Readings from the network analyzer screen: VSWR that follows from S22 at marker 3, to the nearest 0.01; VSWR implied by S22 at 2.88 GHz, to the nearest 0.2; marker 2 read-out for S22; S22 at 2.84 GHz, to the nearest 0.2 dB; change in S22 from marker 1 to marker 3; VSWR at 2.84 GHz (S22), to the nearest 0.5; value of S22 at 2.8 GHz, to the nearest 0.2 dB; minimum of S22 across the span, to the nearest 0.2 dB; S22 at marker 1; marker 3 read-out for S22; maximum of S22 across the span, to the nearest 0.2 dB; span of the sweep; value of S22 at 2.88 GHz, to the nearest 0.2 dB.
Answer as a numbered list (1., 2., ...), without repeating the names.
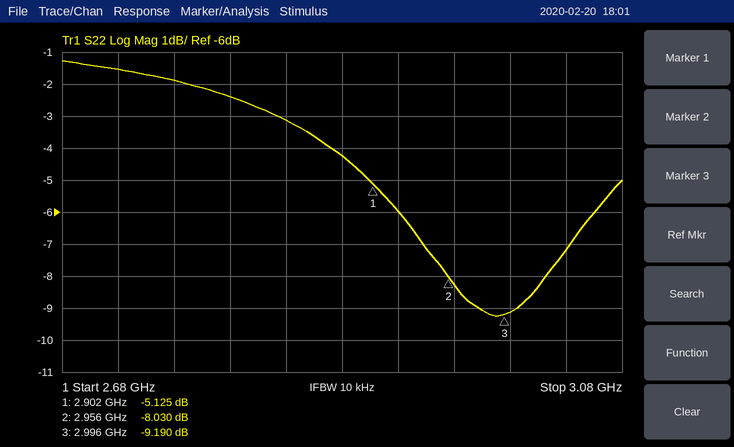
1. 2.06
2. 4.2
3. -8.030 dB
4. -3.2 dB
5. -4.065 dB
6. 5.5
7. -2.4 dB
8. -9.2 dB
9. -5.125 dB
10. -9.190 dB
11. -1.2 dB
12. 400 MHz
13. -4.2 dB
